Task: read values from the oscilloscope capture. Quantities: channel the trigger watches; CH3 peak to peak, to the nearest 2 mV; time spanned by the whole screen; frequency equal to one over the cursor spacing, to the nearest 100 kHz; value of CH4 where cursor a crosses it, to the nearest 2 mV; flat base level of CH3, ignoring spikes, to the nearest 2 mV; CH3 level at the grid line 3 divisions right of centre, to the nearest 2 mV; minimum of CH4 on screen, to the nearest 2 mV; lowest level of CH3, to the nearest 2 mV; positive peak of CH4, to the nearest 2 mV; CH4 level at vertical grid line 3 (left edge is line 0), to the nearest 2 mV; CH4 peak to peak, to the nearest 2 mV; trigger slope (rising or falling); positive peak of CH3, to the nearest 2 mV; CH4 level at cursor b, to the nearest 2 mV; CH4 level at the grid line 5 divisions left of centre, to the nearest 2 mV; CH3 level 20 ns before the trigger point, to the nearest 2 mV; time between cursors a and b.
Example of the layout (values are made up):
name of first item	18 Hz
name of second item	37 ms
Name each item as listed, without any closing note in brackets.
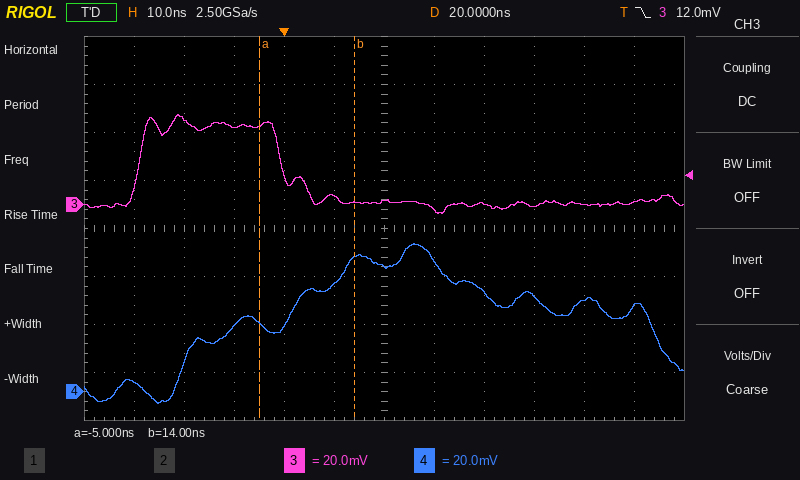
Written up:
channel the trigger watches	CH3
CH3 peak to peak, to the nearest 2 mV	42 mV
time spanned by the whole screen	120 ns
frequency equal to one over the cursor spacing, to the nearest 100 kHz	52.6 MHz
value of CH4 where cursor a crosses it, to the nearest 2 mV	28 mV
flat base level of CH3, ignoring spikes, to the nearest 2 mV	0 mV
CH3 level at the grid line 3 divisions right of centre, to the nearest 2 mV	0 mV
minimum of CH4 on screen, to the nearest 2 mV	-4 mV
lowest level of CH3, to the nearest 2 mV	-4 mV
positive peak of CH4, to the nearest 2 mV	62 mV
CH4 level at vertical grid line 3 (left edge is line 0), to the nearest 2 mV	28 mV
CH4 peak to peak, to the nearest 2 mV	66 mV
trigger slope	falling
positive peak of CH3, to the nearest 2 mV	38 mV
CH4 level at cursor b, to the nearest 2 mV	56 mV
CH4 level at the grid line 5 divisions left of centre, to the nearest 2 mV	4 mV
CH3 level 20 ns before the trigger point, to the nearest 2 mV	36 mV
time between cursors a and b	19 ns
